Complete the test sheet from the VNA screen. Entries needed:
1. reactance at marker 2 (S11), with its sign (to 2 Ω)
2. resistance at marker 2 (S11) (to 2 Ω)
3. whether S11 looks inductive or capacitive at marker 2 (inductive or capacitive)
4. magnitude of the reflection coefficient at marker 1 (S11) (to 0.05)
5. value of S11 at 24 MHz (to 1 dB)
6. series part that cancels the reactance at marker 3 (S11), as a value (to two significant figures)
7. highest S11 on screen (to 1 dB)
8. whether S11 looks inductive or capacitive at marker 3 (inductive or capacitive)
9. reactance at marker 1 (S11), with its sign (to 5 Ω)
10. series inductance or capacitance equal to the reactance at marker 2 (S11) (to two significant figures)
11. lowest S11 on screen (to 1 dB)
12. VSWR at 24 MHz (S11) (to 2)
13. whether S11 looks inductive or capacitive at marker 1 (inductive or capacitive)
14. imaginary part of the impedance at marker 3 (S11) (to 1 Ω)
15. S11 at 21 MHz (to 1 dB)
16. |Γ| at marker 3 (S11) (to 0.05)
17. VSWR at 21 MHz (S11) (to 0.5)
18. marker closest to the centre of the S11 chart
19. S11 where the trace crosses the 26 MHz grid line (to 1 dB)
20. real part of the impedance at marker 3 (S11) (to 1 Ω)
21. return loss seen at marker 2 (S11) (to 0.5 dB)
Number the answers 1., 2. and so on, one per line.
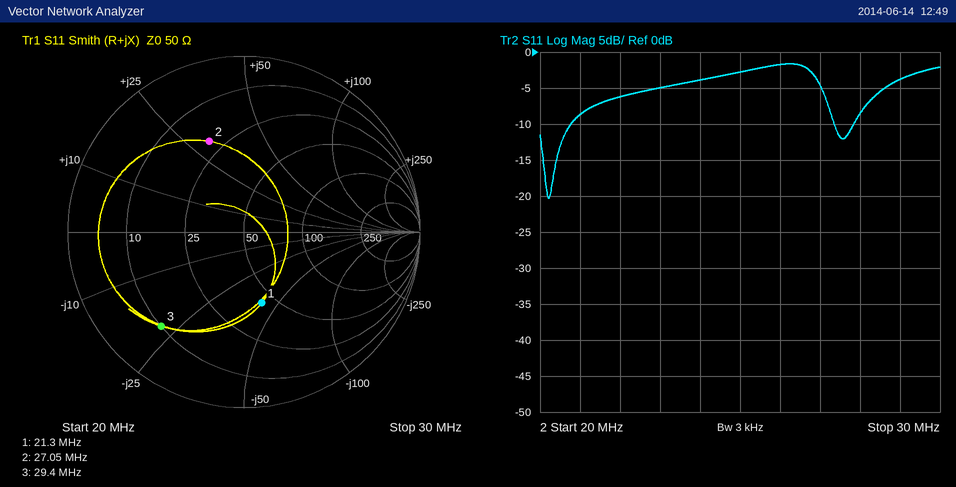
1. +30 Ω
2. 20 Ω
3. inductive
4. 0.40
5. -4 dB
6. 120 nH
7. -2 dB
8. capacitive
9. -40 Ω
10. 180 nH
11. -20 dB
12. 4
13. capacitive
14. -22 Ω
15. -9 dB
16. 0.70
17. 2.0
18. marker 1
19. -2 dB
20. 10 Ω
21. 5.0 dB
